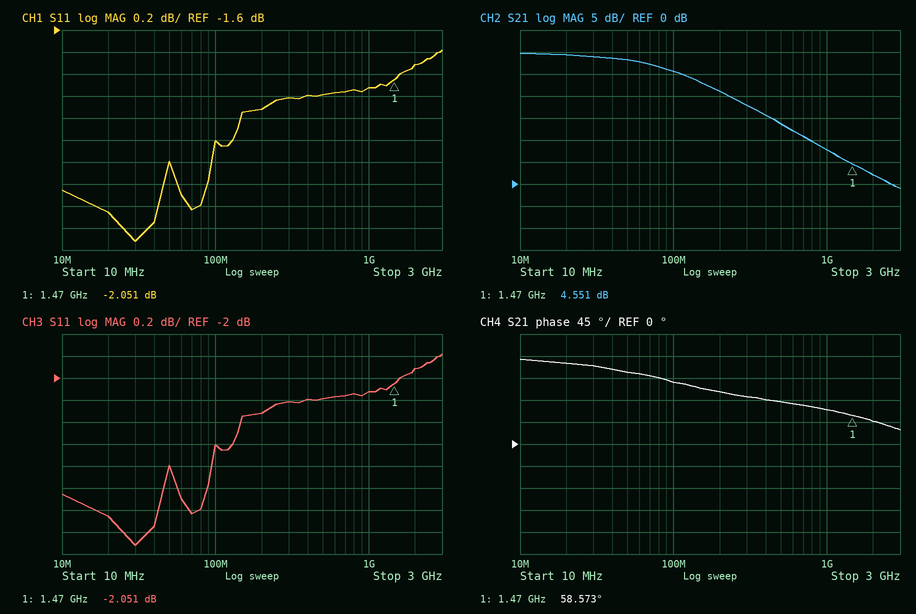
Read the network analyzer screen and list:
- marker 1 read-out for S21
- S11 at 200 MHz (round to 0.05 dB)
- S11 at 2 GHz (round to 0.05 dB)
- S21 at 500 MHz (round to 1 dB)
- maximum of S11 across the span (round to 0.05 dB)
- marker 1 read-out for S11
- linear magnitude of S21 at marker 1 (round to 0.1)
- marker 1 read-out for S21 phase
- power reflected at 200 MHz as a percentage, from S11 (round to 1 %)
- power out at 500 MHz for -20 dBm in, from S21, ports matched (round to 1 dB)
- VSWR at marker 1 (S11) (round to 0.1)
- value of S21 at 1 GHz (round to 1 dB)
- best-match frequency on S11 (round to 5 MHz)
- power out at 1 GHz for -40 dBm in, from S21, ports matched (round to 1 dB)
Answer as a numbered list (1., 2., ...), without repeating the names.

1. 4.551 dB
2. -2.30 dB
3. -1.90 dB
4. 14 dB
5. -1.80 dB
6. -2.051 dB
7. 1.7
8. 58.573°
9. 59 %
10. -6 dBm
11. 8.5
12. 8 dB
13. 30 MHz
14. -32 dBm
